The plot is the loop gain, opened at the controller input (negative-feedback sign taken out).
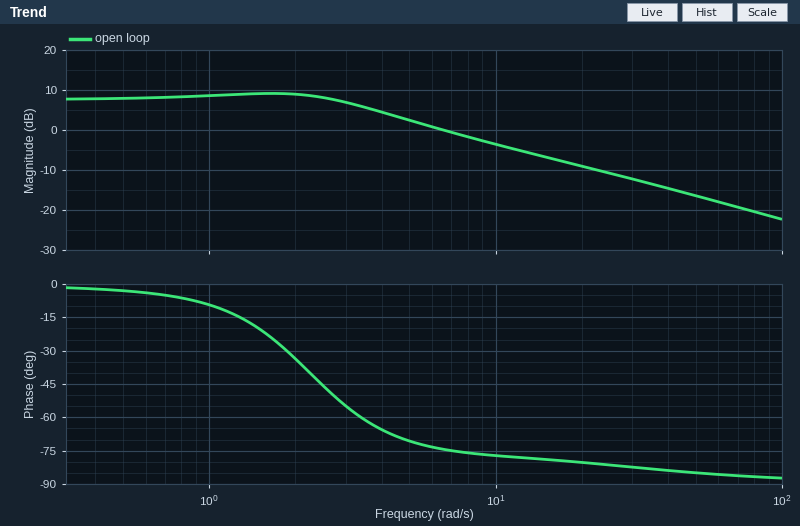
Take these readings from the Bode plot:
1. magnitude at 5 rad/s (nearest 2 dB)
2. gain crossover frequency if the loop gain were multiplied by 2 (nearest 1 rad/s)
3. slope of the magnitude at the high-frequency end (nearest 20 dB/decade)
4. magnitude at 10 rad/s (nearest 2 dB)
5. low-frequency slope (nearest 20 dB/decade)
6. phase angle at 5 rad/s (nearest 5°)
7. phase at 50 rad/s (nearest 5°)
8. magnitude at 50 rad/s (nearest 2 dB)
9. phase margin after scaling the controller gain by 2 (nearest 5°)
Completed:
2 dB
14 rad/s
-20 dB/decade
-4 dB
0 dB/decade
-70°
-85°
-16 dB
100°
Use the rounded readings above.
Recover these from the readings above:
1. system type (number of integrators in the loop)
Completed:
0
